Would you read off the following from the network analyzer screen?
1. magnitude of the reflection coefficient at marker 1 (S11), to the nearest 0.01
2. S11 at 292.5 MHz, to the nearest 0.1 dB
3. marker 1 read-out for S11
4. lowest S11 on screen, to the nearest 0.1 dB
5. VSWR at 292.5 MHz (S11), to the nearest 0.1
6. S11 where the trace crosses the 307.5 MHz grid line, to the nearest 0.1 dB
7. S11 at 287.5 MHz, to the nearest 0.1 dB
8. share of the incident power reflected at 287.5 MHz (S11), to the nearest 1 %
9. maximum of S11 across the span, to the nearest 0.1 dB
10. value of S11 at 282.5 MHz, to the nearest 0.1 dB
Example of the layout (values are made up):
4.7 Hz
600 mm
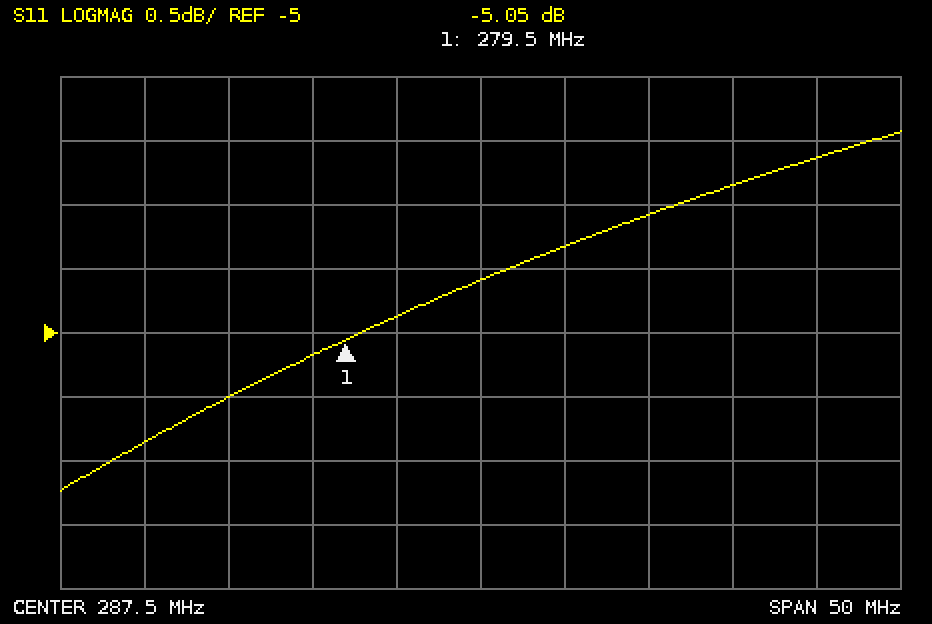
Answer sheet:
0.56
-4.3 dB
-5.05 dB
-6.2 dB
4.1
-3.6 dB
-4.6 dB
35 %
-3.4 dB
-4.9 dB
